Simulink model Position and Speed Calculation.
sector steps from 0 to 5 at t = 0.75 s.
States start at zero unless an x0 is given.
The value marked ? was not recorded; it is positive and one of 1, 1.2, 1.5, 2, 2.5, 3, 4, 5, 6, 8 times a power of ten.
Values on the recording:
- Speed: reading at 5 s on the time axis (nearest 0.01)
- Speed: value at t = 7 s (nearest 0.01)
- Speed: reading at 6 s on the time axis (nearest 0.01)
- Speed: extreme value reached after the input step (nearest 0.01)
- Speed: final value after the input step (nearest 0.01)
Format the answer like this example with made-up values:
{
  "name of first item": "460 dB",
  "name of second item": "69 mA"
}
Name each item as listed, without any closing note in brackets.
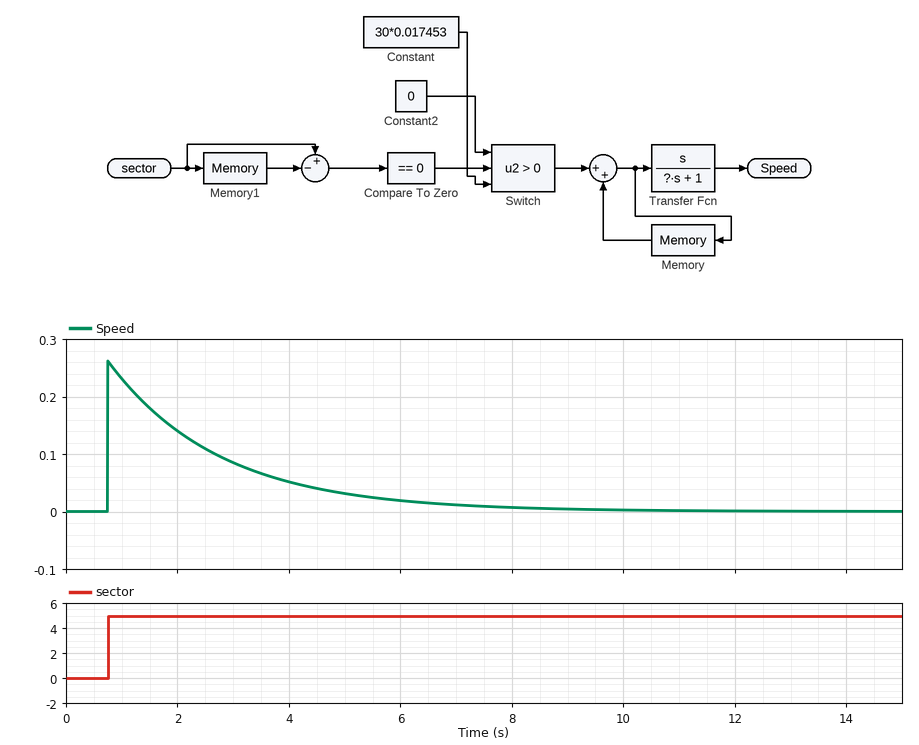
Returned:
{
  "Speed: reading at 5 s on the time axis": "0.03",
  "Speed: value at t = 7 s": "0.01",
  "Speed: reading at 6 s on the time axis": "0.02",
  "Speed: extreme value reached after the input step": "0.26",
  "Speed: final value after the input step": "0.00"
}
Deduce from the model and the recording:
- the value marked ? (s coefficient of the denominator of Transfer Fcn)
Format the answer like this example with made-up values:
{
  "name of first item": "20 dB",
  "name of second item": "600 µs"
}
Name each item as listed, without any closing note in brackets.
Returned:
{
  "the value marked ?": "2"
}
